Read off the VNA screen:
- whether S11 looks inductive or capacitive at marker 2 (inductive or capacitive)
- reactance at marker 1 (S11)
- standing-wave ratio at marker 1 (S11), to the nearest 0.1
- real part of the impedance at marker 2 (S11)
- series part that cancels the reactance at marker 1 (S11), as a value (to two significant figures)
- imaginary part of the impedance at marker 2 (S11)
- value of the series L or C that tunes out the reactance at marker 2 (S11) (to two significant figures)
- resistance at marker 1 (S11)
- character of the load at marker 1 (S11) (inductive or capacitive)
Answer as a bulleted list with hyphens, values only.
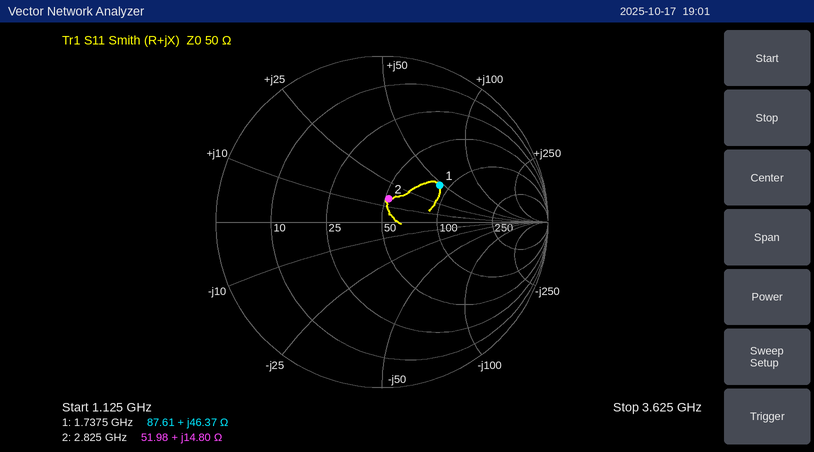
- inductive
- +46.37 Ω
- 2.4
- 51.98 Ω
- 2.0 pF
- +14.80 Ω
- 3.8 pF
- 87.61 Ω
- inductive
